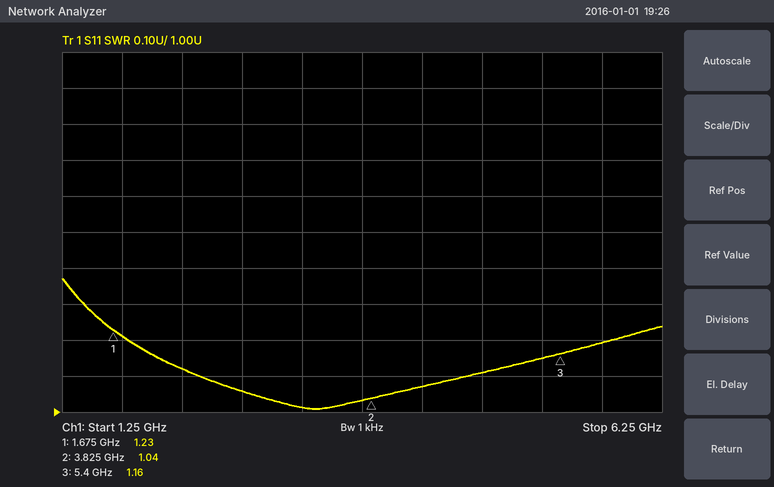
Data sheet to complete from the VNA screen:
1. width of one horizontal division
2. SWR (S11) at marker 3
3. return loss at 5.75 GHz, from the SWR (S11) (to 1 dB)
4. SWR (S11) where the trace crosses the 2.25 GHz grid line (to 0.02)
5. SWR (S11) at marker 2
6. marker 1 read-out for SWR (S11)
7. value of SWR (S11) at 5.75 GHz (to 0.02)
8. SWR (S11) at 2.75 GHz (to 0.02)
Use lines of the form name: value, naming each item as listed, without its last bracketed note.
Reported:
width of one horizontal division: 500 MHz
SWR (S11) at marker 3: 1.16
return loss at 5.75 GHz, from the SWR (S11): 21 dB
SWR (S11) where the trace crosses the 2.25 GHz grid line: 1.12
SWR (S11) at marker 2: 1.04
marker 1 read-out for SWR: 1.23
value of SWR (S11) at 5.75 GHz: 1.20
SWR (S11) at 2.75 GHz: 1.06
